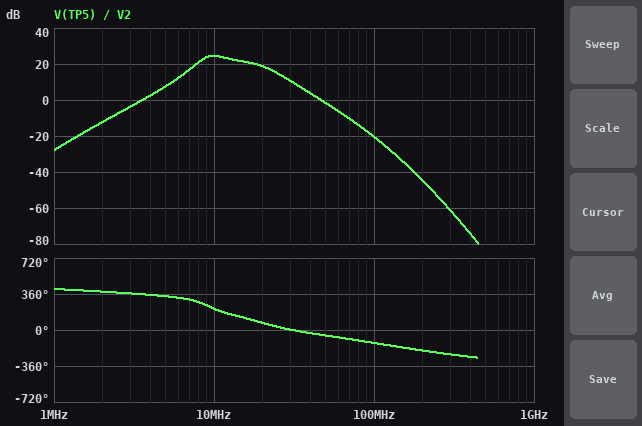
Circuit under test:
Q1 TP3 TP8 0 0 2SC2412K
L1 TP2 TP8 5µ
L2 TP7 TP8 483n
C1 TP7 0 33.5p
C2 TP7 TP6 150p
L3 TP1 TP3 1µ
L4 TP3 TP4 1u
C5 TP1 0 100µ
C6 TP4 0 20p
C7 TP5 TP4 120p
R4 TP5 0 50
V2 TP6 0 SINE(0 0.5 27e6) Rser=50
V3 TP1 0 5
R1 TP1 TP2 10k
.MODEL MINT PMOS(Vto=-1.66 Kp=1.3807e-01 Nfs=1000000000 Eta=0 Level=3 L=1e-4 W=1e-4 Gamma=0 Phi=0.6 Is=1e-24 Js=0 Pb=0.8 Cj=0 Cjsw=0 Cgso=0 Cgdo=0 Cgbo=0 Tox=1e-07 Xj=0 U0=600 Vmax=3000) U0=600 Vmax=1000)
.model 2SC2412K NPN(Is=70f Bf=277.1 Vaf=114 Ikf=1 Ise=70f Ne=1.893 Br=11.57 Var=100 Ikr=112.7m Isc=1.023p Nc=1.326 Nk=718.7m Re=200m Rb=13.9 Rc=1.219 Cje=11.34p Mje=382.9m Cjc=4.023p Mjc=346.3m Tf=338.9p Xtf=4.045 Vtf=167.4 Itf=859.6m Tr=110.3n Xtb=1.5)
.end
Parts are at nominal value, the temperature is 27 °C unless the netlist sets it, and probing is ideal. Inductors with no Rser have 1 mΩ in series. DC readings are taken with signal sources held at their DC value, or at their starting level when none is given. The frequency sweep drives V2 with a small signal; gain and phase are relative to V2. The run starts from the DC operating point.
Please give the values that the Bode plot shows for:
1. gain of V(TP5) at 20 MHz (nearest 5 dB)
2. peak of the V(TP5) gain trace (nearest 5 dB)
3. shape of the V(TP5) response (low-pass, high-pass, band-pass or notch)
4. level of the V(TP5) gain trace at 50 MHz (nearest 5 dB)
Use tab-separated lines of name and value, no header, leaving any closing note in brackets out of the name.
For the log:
gain of V(TP5) at 20 MHz	20 dB
peak of the V(TP5) gain trace	25 dB
shape of the V(TP5) response	band-pass
level of the V(TP5) gain trace at 50 MHz	0 dB
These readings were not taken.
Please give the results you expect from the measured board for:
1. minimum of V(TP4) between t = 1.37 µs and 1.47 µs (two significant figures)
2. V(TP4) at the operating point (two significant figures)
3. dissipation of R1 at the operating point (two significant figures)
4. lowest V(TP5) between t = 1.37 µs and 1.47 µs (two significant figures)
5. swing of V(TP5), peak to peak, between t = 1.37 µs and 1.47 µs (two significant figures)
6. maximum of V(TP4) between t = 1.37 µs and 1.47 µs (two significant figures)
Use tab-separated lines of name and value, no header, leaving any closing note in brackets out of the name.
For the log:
minimum of V(TP4) between t = 1.37 µs and 1.47 µs	2.0 V
V(TP4) at the operating point	5.0 V
dissipation of R1 at the operating point	1.8 mW
lowest V(TP5) between t = 1.37 µs and 1.47 µs	-2.1 V
swing of V(TP5), peak to peak, between t = 1.37 µs and 1.47 µs	4.2 V
maximum of V(TP4) between t = 1.37 µs and 1.47 µs	7.8 V
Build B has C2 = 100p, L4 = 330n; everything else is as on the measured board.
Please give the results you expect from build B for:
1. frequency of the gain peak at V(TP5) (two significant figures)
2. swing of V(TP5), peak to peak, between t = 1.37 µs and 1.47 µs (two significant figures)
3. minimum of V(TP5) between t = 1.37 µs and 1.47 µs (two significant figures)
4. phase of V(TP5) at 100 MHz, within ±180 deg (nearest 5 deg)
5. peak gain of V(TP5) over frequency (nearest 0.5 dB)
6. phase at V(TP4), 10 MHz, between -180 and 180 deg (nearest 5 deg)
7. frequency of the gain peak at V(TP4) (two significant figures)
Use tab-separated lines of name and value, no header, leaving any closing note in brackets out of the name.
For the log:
frequency of the gain peak at V(TP5)	13 MHz
swing of V(TP5), peak to peak, between t = 1.37 µs and 1.47 µs	7.7 V
minimum of V(TP5) between t = 1.37 µs and 1.47 µs	-3.6 V
phase of V(TP5) at 100 MHz, within ±180 deg	-100 deg
peak gain of V(TP5) over frequency	23.0 dB
phase at V(TP4), 10 MHz, between -180 and 180 deg	-165 deg
frequency of the gain peak at V(TP4)	12 MHz
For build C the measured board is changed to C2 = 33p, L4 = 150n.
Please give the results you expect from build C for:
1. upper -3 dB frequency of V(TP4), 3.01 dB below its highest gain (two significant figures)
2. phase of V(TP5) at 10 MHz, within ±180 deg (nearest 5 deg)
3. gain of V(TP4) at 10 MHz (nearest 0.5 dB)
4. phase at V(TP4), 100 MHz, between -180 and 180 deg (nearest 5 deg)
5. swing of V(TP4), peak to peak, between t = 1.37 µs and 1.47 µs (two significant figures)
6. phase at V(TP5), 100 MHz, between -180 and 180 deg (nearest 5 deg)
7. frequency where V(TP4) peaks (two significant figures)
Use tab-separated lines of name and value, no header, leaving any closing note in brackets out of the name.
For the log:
upper -3 dB frequency of V(TP4), 3.01 dB below its highest gain	32 MHz
phase of V(TP5) at 10 MHz, within ±180 deg	-70 deg
gain of V(TP4) at 10 MHz	19.0 dB
phase at V(TP4), 100 MHz, between -180 and 180 deg	-80 deg
swing of V(TP4), peak to peak, between t = 1.37 µs and 1.47 µs	12 V
phase at V(TP5), 100 MHz, between -180 and 180 deg	-65 deg
frequency where V(TP4) peaks	28 MHz
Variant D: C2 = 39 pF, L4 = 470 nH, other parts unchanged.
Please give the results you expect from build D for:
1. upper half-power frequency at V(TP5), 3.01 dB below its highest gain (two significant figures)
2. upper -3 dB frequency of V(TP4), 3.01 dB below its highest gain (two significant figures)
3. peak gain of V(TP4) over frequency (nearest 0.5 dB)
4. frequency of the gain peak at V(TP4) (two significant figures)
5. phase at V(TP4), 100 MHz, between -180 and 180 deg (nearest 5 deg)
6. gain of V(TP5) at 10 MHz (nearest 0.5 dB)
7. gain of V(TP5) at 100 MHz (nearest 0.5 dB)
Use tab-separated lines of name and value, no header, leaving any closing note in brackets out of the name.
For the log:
upper half-power frequency at V(TP5), 3.01 dB below its highest gain	32 MHz
upper -3 dB frequency of V(TP4), 3.01 dB below its highest gain	30 MHz
peak gain of V(TP4) over frequency	22.5 dB
frequency of the gain peak at V(TP4)	11 MHz
phase at V(TP4), 100 MHz, between -180 and 180 deg	-115 deg
gain of V(TP5) at 10 MHz	12.5 dB
gain of V(TP5) at 100 MHz	-17.5 dB
